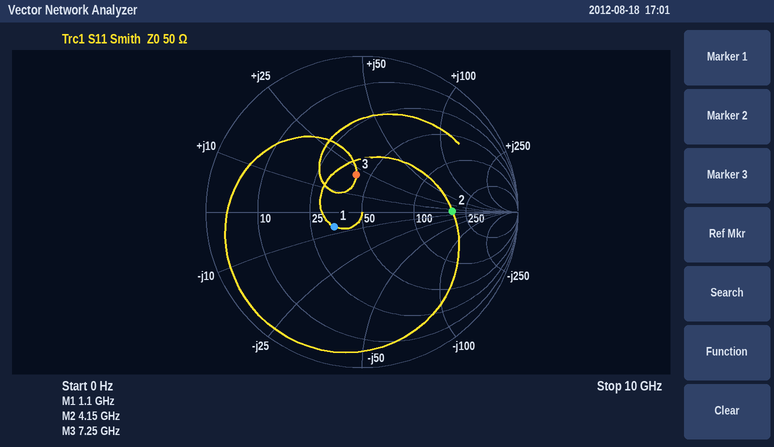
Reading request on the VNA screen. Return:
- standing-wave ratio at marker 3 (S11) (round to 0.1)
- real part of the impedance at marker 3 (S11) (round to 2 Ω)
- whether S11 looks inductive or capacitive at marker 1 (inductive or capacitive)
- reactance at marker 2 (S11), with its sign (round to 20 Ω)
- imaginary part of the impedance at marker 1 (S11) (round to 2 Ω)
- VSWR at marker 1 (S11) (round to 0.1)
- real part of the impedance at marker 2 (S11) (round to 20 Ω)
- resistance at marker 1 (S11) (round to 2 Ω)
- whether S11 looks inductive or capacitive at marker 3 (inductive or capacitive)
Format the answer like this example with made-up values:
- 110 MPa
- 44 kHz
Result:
- 1.6
- 42 Ω
- capacitive
- 0 Ω
- -6 Ω
- 1.5
- 180 Ω
- 34 Ω
- inductive
